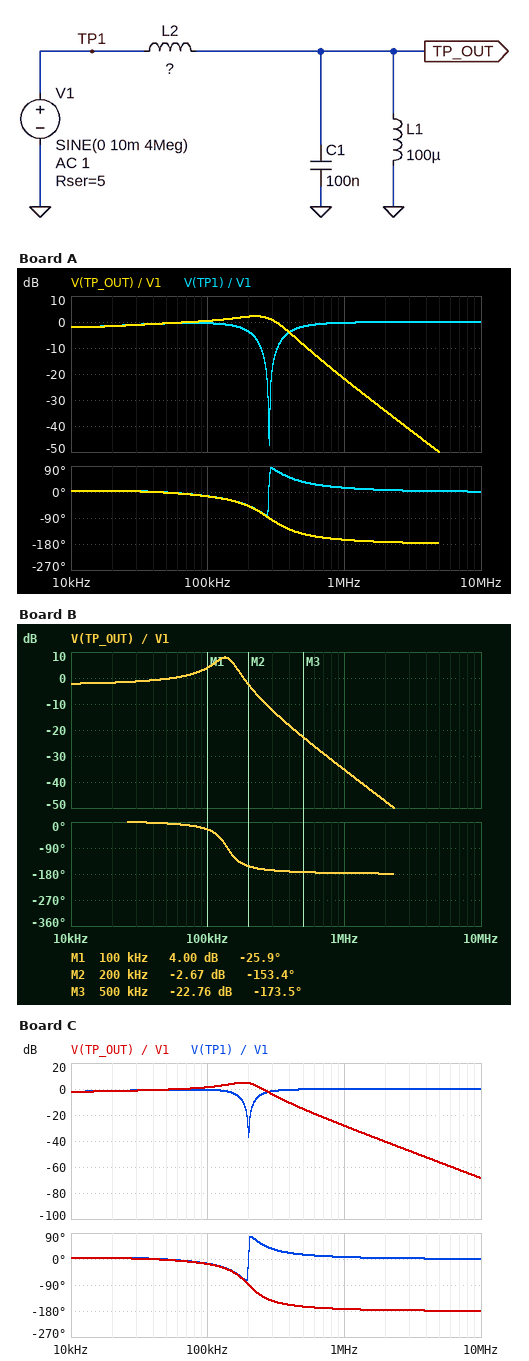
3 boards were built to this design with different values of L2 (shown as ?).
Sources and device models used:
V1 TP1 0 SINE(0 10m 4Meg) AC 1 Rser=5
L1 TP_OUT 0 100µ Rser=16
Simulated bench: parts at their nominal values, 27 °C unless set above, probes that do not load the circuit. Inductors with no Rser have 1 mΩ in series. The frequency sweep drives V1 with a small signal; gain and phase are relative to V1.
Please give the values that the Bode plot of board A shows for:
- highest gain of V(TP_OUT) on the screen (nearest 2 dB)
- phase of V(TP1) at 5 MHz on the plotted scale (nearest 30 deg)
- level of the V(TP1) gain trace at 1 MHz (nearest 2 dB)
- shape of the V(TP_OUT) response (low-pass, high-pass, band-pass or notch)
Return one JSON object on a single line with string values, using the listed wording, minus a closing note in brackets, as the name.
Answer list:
{"highest gain of V(TP_OUT) on the screen": "2 dB", "phase of V(TP1) at 5 MHz on the plotted scale": "0 deg", "level of the V(TP1) gain trace at 1 MHz": "0 dB", "shape of the V(TP_OUT) response": "low-pass"}
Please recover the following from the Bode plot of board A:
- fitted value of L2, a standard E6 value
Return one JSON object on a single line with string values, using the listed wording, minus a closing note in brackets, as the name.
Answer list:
{"fitted value of L2, a standard E6 value": "3.3 µH"}
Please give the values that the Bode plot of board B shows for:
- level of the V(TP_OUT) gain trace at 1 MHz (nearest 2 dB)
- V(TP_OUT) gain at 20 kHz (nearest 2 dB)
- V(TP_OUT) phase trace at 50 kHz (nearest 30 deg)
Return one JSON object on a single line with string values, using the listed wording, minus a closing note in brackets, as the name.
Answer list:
{"level of the V(TP_OUT) gain trace at 1 MHz": "-36 dB", "V(TP_OUT) gain at 20 kHz": "-2 dB", "V(TP_OUT) phase trace at 50 kHz": "0 deg"}
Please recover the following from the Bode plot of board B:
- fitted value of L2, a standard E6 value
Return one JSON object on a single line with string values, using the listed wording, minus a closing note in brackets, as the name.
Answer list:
{"fitted value of L2, a standard E6 value": "15 µH"}
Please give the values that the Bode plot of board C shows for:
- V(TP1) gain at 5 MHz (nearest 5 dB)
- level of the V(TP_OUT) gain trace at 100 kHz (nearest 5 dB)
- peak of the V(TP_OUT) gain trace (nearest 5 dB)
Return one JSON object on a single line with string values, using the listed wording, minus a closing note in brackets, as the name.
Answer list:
{"V(TP1) gain at 5 MHz": "0 dB", "level of the V(TP_OUT) gain trace at 100 kHz": "0 dB", "peak of the V(TP_OUT) gain trace": "5 dB"}
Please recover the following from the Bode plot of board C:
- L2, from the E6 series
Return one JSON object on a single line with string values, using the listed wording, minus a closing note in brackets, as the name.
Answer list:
{"L2, from the E6 series": "6.8 µH"}
